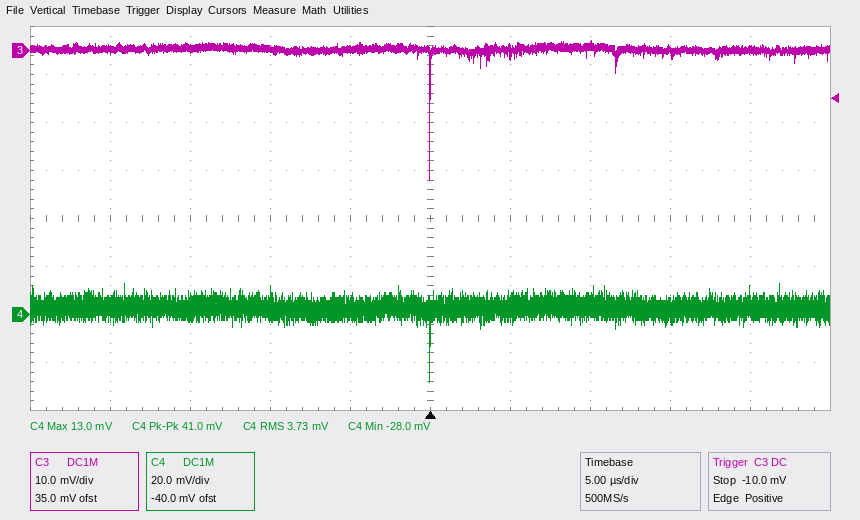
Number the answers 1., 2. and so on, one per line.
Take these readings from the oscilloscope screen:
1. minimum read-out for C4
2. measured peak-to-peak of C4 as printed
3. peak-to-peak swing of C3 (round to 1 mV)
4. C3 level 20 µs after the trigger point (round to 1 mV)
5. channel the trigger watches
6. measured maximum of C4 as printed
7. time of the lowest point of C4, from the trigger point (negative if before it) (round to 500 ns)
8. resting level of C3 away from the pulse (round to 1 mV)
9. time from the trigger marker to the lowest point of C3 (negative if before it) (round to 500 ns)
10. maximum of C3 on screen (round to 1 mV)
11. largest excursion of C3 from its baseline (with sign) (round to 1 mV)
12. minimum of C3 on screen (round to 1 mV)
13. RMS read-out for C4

1. -28.0 mV
2. 41.0 mV
3. 29 mV
4. 0 mV
5. C3
6. 13.0 mV
7. 0.0 µs
8. 0 mV
9. 0.0 µs
10. 2 mV
11. -27 mV
12. -27 mV
13. 3.73 mV
